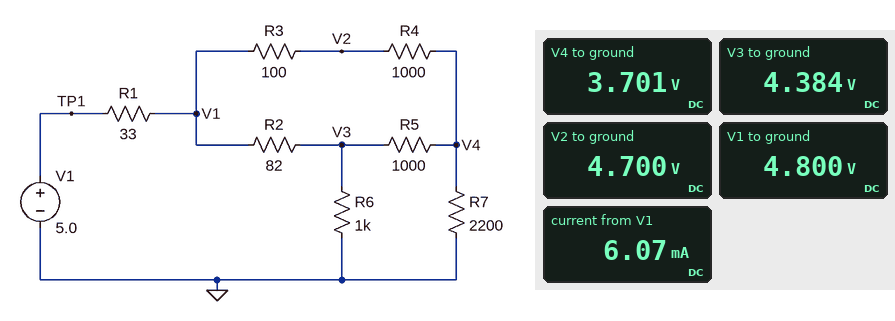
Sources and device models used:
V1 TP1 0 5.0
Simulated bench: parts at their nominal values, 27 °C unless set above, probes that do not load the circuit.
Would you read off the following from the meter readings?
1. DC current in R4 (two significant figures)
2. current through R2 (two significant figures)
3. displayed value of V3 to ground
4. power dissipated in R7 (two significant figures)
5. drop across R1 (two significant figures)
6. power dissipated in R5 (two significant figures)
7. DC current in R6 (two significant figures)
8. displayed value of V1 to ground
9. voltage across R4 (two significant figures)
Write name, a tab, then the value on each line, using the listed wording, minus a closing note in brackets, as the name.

DC current in R4	1.0 mA
current through R2	5.1 mA
displayed value of V3 to ground	4.384 V
power dissipated in R7	6.2 mW
drop across R1	200 mV
power dissipated in R5	470 µW
DC current in R6	4.4 mA
displayed value of V1 to ground	4.800 V
voltage across R4	1.0 V
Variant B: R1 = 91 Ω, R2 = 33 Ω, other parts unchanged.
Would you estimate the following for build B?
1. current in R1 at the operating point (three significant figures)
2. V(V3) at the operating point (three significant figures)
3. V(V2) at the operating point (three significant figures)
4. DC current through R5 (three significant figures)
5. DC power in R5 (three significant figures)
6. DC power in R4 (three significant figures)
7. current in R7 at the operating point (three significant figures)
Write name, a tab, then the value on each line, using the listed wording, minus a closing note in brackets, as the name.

current in R1 at the operating point	5.90 mA
V(V3) at the operating point	4.30 V
V(V2) at the operating point	4.38 V
DC current through R5	762 µA
DC power in R5	581 µW
DC power in R4	713 µW
current in R7 at the operating point	1.61 mA
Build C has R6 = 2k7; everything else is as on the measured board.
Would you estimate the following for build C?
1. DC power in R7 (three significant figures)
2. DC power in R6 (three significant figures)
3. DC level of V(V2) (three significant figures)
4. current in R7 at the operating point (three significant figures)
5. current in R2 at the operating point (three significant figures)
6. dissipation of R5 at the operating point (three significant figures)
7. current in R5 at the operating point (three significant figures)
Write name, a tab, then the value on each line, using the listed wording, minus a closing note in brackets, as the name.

DC power in R7	6.76 mW
DC power in R6	8.10 mW
DC level of V(V2)	4.79 V
current in R7 at the operating point	1.75 mA
current in R2 at the operating point	2.55 mA
dissipation of R5 at the operating point	670 µW
current in R5 at the operating point	819 µA
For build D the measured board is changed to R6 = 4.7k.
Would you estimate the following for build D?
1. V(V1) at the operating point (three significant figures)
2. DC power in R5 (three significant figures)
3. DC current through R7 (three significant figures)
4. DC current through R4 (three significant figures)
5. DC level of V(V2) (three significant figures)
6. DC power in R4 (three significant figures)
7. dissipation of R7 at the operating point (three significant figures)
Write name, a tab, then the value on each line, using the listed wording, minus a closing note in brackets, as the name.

V(V1) at the operating point	4.91 V
DC power in R5	732 µW
DC current through R7	1.77 mA
DC current through R4	917 µA
DC level of V(V2)	4.82 V
DC power in R4	841 µW
dissipation of R7 at the operating point	6.91 mW
